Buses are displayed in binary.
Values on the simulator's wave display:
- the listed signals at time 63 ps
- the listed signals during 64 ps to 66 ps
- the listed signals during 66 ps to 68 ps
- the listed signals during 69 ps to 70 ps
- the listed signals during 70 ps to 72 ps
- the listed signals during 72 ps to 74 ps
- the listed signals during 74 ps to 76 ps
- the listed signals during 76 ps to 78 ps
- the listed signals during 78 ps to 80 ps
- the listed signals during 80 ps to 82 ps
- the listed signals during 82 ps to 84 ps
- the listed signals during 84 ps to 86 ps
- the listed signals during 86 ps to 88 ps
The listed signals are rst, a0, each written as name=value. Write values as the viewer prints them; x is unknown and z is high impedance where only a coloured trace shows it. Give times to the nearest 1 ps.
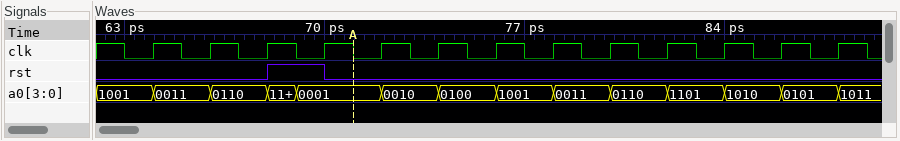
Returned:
rst=0, a0=1001
rst=0, a0=0011
rst=0, a0=0110
rst=1, a0=0001
rst=0, a0=0001
rst=0, a0=0010
rst=0, a0=0100
rst=0, a0=1001
rst=0, a0=0011
rst=0, a0=0110
rst=0, a0=1101
rst=0, a0=1010
rst=0, a0=0101
